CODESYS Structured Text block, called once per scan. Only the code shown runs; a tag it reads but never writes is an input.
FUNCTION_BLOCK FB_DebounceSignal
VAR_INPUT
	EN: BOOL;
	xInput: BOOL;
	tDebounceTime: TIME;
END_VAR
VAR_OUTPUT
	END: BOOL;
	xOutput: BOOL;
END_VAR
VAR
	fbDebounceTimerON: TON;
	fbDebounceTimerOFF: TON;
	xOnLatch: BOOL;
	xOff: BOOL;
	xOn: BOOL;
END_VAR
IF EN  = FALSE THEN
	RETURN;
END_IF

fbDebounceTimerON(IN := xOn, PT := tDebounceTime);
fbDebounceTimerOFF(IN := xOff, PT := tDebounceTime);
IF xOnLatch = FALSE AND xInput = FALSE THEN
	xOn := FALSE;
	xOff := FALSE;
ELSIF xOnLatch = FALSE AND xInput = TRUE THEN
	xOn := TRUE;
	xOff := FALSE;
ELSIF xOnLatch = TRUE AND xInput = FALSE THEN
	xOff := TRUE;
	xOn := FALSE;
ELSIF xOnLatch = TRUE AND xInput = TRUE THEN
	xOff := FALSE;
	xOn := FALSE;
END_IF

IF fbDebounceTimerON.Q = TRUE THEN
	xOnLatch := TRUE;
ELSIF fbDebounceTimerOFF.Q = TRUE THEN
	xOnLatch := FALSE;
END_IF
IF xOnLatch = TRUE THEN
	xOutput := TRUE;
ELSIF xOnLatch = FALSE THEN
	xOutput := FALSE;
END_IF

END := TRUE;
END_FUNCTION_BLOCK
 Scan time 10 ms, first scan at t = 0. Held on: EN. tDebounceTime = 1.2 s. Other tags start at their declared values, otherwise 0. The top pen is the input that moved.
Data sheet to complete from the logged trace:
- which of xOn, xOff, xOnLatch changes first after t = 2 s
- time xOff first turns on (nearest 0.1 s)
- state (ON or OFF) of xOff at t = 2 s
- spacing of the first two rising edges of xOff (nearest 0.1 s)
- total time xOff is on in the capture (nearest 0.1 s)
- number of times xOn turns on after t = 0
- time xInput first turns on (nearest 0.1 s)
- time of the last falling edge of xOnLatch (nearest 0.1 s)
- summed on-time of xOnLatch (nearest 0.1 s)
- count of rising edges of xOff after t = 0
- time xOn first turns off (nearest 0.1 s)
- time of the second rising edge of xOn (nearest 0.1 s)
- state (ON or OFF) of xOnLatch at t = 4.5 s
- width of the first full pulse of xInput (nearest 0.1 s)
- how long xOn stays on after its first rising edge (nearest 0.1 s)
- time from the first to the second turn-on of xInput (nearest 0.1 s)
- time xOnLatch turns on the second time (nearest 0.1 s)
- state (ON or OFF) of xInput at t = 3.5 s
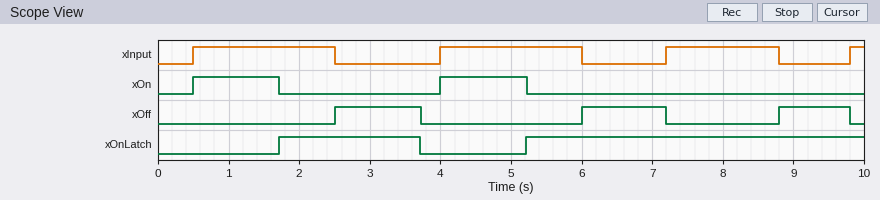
xOff
2.5 s
OFF
3.5 s
3.4 s
2
0.5 s
3.7 s
6.8 s
3
1.7 s
4.0 s
OFF
2.0 s
1.2 s
3.5 s
5.2 s
OFF
